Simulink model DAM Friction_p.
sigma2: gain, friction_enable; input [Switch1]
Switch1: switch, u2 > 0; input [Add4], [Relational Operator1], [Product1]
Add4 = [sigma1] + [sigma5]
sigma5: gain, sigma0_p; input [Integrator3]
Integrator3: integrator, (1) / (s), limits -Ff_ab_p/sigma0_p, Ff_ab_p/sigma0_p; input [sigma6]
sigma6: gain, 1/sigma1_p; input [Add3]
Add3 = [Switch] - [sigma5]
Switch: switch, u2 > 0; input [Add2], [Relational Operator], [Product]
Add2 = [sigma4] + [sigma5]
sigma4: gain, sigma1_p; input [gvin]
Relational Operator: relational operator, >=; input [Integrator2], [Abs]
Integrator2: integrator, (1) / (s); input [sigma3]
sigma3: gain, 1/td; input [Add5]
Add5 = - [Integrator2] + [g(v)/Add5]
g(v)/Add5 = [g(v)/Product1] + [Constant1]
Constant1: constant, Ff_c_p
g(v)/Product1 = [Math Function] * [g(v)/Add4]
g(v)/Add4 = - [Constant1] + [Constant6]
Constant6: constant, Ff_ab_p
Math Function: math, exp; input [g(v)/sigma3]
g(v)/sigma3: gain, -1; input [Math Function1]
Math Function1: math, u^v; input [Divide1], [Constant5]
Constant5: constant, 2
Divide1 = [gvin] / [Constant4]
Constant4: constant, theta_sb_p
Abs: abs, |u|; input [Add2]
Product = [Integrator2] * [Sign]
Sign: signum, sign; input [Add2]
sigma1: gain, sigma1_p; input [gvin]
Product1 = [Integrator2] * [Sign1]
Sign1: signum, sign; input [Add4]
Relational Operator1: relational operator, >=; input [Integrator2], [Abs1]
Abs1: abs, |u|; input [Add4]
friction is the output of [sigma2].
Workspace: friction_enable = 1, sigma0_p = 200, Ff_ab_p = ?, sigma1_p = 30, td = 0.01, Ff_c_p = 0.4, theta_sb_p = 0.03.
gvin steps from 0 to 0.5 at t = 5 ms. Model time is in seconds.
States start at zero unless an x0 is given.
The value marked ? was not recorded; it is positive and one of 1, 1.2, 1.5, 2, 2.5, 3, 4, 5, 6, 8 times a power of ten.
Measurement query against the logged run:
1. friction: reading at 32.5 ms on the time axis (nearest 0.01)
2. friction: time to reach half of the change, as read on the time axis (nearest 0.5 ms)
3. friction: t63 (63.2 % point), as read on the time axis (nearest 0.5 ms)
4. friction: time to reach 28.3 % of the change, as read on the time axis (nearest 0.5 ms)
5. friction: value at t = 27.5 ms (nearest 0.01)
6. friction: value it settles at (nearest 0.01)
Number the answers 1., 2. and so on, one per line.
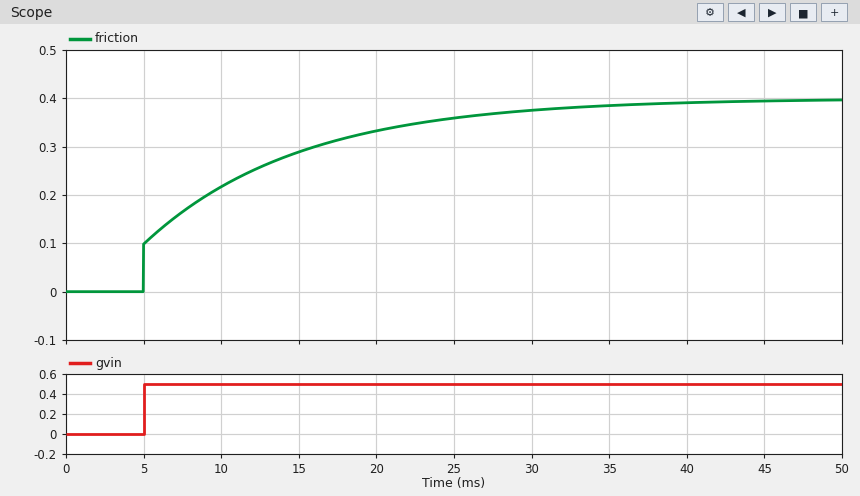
1. 0.38
2. 9.0 ms
3. 12.0 ms
4. 5.5 ms
5. 0.37
6. 0.40
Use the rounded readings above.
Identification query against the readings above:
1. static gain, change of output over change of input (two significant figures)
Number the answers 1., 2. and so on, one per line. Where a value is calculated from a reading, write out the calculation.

1. (0.4 - 0) / (0.5 - 0) = 0.80
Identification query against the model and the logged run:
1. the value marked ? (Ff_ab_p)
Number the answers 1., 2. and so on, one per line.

1. 0.25
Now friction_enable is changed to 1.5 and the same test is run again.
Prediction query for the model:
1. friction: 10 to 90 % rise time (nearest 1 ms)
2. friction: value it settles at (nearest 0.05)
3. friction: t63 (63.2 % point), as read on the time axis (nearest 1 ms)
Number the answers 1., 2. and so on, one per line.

1. 20 ms
2. 0.60
3. 12 ms
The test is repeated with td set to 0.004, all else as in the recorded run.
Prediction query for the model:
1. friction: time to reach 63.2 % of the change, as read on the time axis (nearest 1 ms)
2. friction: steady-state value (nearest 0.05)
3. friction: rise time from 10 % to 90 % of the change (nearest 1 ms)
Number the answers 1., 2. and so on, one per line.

1. 7 ms
2. 0.40
3. 7 ms
